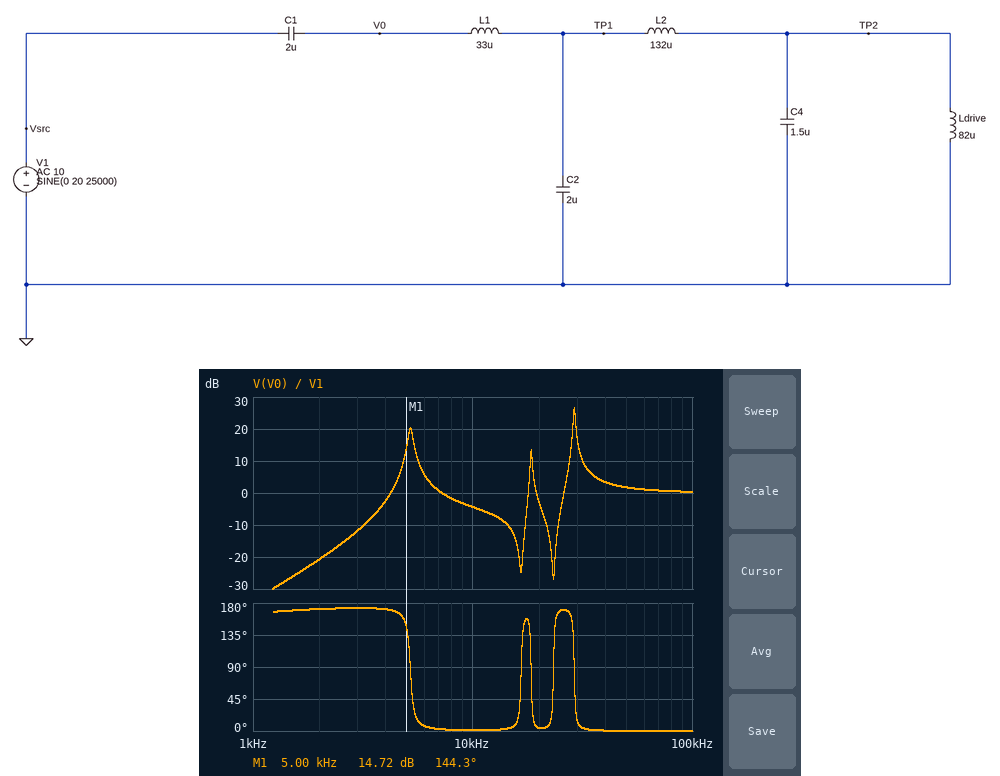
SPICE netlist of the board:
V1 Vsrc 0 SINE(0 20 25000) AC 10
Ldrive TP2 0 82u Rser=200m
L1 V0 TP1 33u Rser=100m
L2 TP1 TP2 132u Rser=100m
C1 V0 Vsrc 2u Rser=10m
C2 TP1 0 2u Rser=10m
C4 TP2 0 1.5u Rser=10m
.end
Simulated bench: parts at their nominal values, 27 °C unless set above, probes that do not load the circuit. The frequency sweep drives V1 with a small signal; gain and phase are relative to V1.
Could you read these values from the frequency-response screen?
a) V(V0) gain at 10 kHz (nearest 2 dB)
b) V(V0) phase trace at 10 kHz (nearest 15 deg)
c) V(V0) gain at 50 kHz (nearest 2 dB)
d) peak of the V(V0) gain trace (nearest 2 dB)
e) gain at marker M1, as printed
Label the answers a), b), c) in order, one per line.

a) -4 dB
b) 0 deg
c) 2 dB
d) 26 dB
e) 14.72 dB
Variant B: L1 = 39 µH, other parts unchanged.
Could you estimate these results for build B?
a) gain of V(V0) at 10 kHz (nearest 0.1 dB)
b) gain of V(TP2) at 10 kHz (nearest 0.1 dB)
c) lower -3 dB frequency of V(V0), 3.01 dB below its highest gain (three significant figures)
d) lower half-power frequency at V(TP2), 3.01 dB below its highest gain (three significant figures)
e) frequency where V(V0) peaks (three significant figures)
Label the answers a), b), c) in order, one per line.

a) -4.5 dB
b) -8.1 dB
c) 26.6 kHz
d) 18.1 kHz
e) 26.8 kHz
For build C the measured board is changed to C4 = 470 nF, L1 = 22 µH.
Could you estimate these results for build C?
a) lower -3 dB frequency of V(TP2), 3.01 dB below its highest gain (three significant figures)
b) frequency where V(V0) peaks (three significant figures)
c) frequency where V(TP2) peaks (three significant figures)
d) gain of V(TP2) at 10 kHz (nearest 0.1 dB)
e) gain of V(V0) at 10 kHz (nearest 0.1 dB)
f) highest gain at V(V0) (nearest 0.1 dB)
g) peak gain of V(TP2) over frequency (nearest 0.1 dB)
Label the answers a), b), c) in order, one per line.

a) 31.2 kHz
b) 36.1 kHz
c) 31.4 kHz
d) -10.2 dB
e) -3.4 dB
f) 23.5 dB
g) 33.5 dB
